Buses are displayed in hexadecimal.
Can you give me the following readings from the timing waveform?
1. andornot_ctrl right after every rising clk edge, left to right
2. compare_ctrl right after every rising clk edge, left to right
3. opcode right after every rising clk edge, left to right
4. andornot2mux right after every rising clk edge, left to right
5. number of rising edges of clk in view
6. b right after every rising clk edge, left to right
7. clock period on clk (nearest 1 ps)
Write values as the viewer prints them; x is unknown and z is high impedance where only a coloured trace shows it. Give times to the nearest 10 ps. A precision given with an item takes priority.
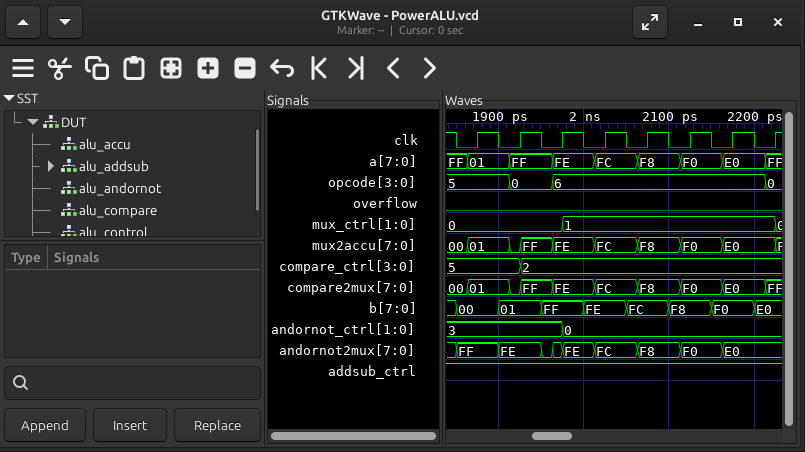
3, 3, 0, 0, 0, 0, 0, 0
5, 2, 2, 2, 2, 2, 2, 2
5, 0, 6, 6, 6, 6, 6, 0
FF, FE, FE, FC, F8, F0, E0, E0
8
00, 01, FF, FE, FC, F8, F0, E0
50 ps
